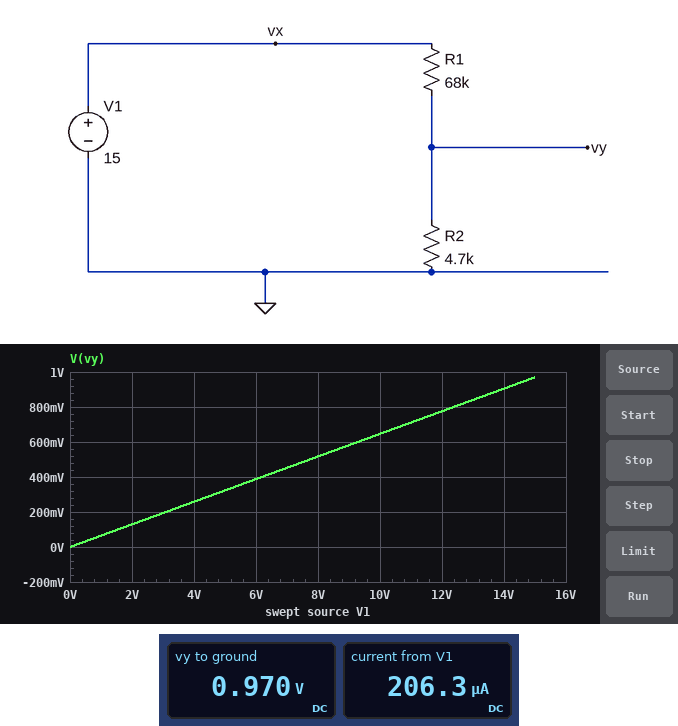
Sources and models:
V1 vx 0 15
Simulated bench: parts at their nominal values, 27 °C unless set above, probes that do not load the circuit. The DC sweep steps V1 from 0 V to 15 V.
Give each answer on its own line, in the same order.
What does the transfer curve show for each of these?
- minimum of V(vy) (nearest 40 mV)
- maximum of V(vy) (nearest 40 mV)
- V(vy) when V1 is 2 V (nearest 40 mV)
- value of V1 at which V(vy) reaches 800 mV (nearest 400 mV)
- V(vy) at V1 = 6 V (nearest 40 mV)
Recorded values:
0 V
960 mV
120 mV
12.4 V
400 mV
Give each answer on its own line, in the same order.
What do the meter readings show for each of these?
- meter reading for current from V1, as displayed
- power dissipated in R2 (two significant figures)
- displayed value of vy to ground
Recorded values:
206.3 µA
200 µW
0.970 V
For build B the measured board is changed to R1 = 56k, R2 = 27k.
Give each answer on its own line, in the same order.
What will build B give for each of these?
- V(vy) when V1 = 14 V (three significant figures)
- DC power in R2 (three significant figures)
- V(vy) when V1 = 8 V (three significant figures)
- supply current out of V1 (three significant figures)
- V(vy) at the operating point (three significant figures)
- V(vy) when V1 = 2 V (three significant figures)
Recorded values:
4.55 V
882 µW
2.60 V
181 µA
4.88 V
651 mV
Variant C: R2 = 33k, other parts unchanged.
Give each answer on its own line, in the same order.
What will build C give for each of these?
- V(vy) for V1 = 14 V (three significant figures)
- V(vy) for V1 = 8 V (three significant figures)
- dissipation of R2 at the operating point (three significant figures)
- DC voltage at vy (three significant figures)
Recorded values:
4.57 V
2.61 V
728 µW
4.90 V
